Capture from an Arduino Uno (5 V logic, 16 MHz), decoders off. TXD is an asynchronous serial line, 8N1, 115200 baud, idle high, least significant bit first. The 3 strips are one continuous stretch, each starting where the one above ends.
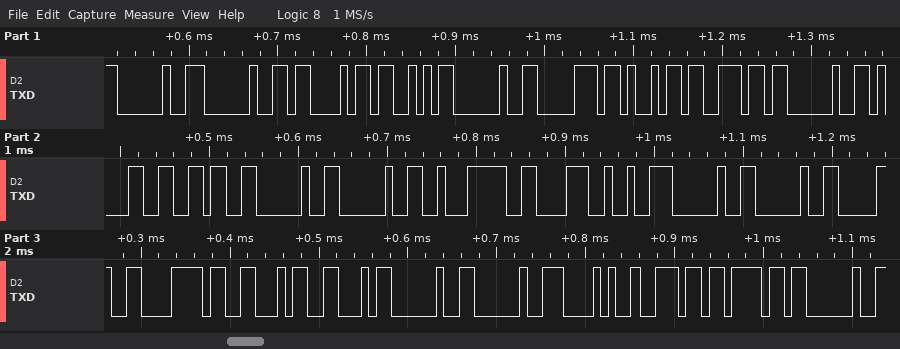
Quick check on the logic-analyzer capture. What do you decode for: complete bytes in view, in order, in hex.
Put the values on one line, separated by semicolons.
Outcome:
20 20 43 53 20 70 69 6E 20 31 36 20 20 E2 86 92 20 20 30 78 46 46 20 20 28 6E 6F 20
